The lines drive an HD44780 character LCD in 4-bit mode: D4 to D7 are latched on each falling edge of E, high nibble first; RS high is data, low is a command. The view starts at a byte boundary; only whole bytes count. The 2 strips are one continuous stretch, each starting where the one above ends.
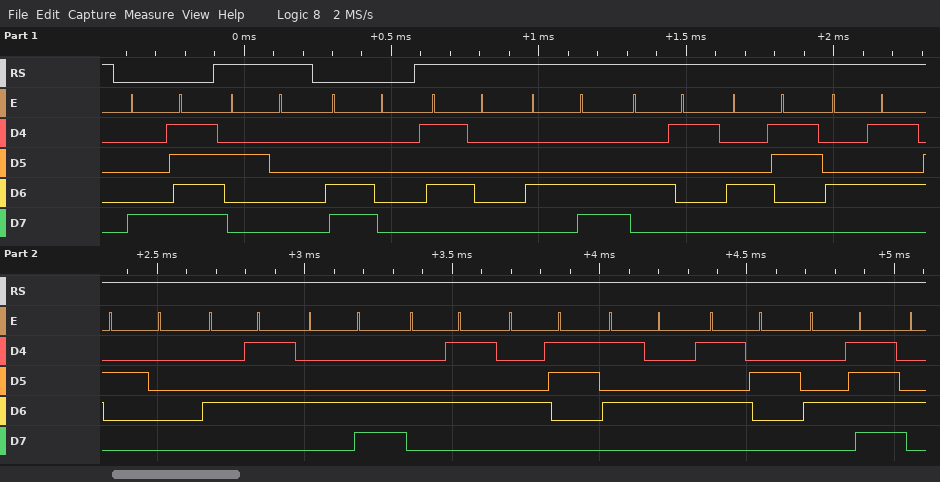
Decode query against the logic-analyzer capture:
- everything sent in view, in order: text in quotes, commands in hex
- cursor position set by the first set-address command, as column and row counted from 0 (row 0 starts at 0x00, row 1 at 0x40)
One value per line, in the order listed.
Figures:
0x8F " " 0xC0 "PLACE ELECTRO"
column 15, row 0
